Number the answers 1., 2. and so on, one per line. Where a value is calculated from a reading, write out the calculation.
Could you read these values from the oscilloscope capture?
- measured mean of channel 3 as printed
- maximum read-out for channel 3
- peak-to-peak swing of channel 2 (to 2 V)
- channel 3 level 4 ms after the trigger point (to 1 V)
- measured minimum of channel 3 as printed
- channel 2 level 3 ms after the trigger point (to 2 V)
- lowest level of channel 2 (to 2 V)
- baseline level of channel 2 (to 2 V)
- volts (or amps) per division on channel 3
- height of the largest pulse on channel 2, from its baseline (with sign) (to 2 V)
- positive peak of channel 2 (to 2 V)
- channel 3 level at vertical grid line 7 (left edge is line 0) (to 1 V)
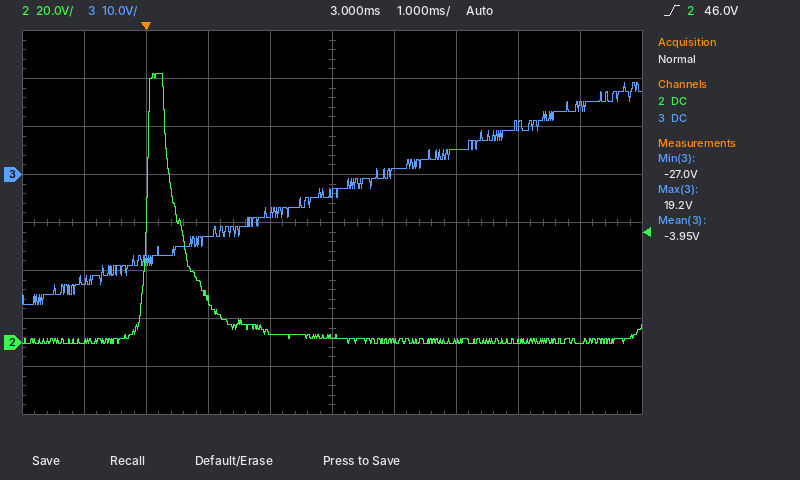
1. -3.95 V
2. 19.2 V
3. 112 V − (0 V) = 112 V
4. 1 V
5. -27.0 V
6. 2 V
7. 0 V
8. 0 V
9. 10 V
10. 112 V − (0 V) = +112 V
11. 112 V
12. 5 V
